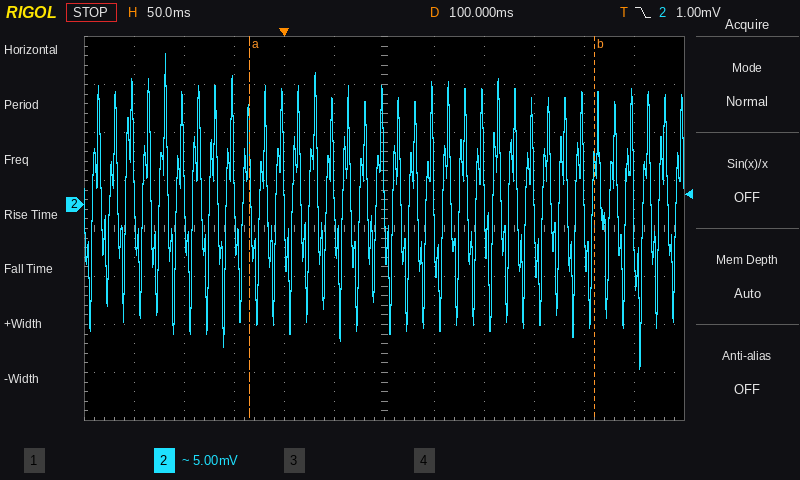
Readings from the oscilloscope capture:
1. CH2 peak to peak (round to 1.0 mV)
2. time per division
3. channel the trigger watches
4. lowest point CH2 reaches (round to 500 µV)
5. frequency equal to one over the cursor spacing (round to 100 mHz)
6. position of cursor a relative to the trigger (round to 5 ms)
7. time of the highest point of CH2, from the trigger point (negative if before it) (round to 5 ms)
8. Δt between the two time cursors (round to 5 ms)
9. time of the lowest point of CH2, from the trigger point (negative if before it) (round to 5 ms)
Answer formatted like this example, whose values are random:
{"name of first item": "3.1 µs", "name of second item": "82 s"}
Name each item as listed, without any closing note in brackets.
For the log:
{"CH2 peak to peak": "33.0 mV", "time per division": "50 ms", "channel the trigger watches": "CH2", "lowest point CH2 reaches": "-17.0 mV", "frequency equal to one over the cursor spacing": "2.9 Hz", "position of cursor a relative to the trigger": "-35 ms", "time of the highest point of CH2, from the trigger point (negative if before it)": "-120 ms", "Δt between the two time cursors": "345 ms", "time of the lowest point of CH2, from the trigger point (negative if before it)": "+355 ms"}
